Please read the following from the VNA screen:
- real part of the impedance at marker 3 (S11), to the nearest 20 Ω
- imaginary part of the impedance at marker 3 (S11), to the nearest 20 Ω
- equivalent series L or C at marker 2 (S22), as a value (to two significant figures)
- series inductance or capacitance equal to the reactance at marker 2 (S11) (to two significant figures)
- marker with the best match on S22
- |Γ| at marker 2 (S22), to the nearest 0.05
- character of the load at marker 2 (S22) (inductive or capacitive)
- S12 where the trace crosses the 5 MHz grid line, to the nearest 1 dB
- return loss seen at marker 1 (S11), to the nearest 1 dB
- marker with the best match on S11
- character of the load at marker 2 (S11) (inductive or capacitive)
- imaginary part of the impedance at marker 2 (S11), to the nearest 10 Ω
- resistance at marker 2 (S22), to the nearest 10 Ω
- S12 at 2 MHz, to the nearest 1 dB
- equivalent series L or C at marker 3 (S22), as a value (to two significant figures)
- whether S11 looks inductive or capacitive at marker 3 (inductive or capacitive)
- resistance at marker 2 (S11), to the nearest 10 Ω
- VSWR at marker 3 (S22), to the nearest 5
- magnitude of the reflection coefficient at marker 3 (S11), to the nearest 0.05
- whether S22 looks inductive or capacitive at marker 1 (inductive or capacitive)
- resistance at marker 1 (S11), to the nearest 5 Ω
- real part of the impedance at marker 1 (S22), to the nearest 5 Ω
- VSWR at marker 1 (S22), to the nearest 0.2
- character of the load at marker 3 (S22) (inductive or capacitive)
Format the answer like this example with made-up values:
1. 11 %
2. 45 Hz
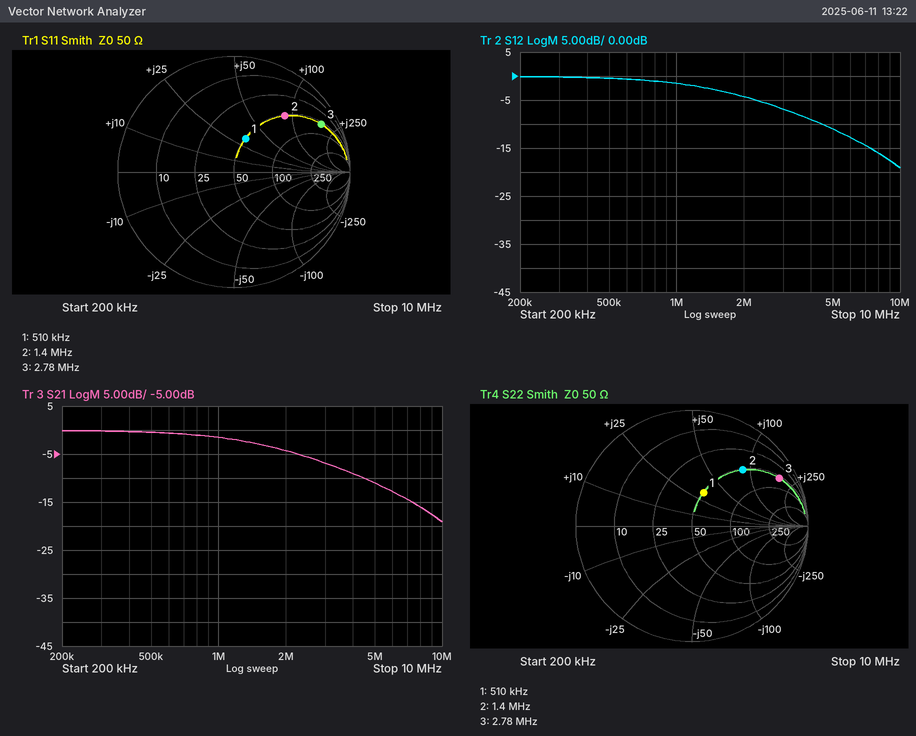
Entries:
1. 60 Ω
2. +180 Ω
3. 10 µH
4. 10 µH
5. marker 1
6. 0.65
7. inductive
8. -11 dB
9. 10 dB
10. marker 1
11. inductive
12. +90 Ω
13. 50 Ω
14. -4 dB
15. 10 µH
16. inductive
17. 50 Ω
18. 15
19. 0.85
20. inductive
21. 50 Ω
22. 50 Ω
23. 1.8
24. inductive
